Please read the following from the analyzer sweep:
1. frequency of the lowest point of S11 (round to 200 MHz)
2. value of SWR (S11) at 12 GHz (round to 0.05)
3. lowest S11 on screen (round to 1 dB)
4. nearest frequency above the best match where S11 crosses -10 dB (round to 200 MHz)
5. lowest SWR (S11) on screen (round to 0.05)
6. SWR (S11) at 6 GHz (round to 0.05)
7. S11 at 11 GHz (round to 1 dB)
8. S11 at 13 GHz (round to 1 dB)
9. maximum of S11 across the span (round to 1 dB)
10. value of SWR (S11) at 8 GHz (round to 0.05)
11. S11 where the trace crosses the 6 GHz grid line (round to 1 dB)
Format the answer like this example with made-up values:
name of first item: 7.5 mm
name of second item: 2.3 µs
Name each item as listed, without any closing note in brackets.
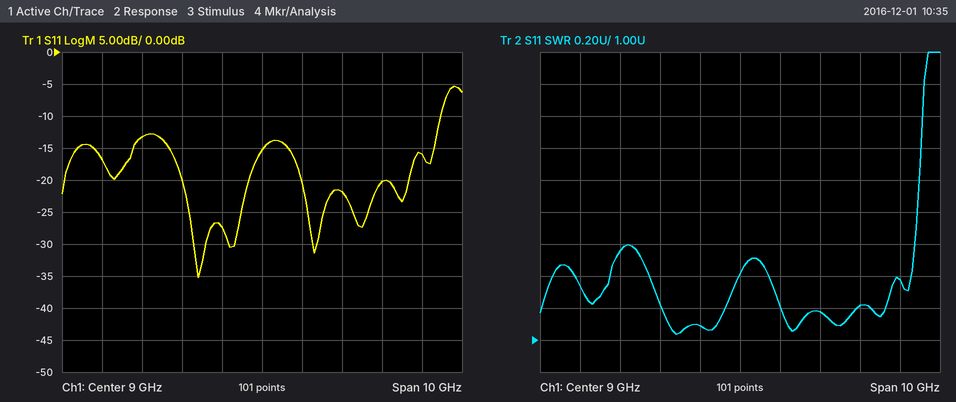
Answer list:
frequency of the lowest point of S11: 7.4 GHz
value of SWR (S11) at 12 GHz: 1.20
lowest S11 on screen: -35 dB
nearest frequency above the best match where S11 crosses -10 dB: 13.4 GHz
lowest SWR (S11) on screen: 1.05
SWR (S11) at 6 GHz: 1.55
S11 at 11 GHz: -22 dB
S11 at 13 GHz: -16 dB
maximum of S11 across the span: -5 dB
value of SWR (S11) at 8 GHz: 1.10
S11 where the trace crosses the 6 GHz grid line: -13 dB
